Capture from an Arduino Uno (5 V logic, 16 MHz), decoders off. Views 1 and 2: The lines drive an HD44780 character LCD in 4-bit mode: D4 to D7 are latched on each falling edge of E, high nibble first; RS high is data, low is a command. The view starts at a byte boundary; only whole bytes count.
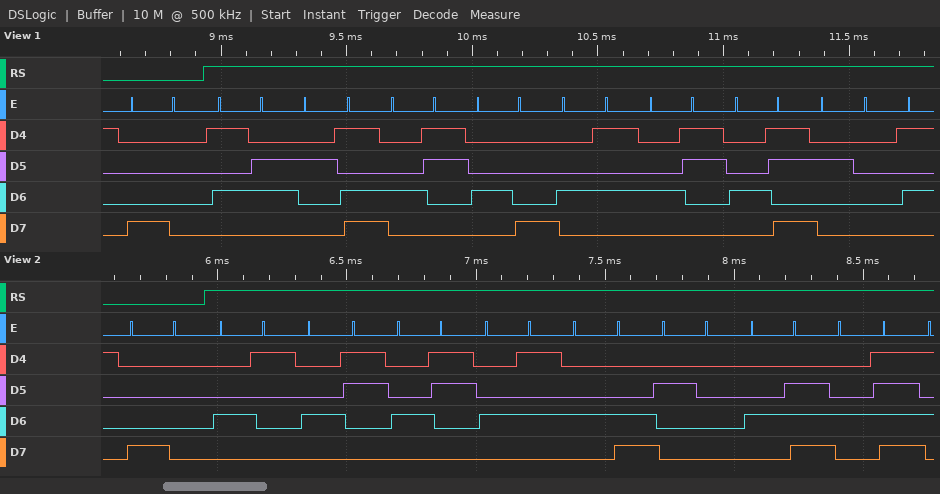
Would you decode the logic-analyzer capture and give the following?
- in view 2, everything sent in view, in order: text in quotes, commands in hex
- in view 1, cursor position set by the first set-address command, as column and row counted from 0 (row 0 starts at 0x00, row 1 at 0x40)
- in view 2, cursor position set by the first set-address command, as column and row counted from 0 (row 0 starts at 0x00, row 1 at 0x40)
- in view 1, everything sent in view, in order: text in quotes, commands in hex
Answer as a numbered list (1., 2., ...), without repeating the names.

1. 0x80 "ACCEL NO"
2. column 0, row 0
3. column 0, row 0
4. 0x80 "V-CHECK "
